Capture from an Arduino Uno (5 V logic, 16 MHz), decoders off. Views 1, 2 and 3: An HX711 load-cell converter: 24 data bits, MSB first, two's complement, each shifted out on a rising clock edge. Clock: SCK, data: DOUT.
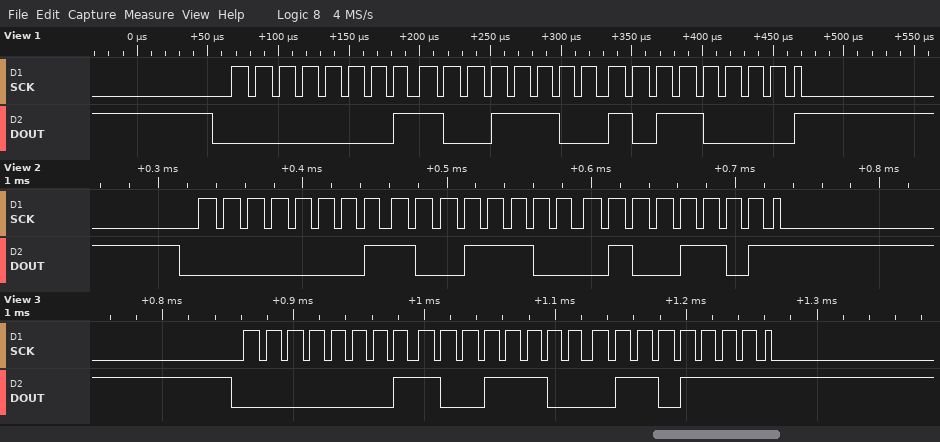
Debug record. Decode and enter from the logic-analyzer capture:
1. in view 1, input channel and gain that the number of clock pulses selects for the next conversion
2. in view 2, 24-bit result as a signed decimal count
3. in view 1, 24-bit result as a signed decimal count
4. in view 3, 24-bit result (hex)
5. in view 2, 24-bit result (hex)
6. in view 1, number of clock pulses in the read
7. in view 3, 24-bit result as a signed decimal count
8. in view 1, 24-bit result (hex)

channel A, gain 128
105549
105648
0x019C6F
0x019C4D
25
105583
0x019CB0
